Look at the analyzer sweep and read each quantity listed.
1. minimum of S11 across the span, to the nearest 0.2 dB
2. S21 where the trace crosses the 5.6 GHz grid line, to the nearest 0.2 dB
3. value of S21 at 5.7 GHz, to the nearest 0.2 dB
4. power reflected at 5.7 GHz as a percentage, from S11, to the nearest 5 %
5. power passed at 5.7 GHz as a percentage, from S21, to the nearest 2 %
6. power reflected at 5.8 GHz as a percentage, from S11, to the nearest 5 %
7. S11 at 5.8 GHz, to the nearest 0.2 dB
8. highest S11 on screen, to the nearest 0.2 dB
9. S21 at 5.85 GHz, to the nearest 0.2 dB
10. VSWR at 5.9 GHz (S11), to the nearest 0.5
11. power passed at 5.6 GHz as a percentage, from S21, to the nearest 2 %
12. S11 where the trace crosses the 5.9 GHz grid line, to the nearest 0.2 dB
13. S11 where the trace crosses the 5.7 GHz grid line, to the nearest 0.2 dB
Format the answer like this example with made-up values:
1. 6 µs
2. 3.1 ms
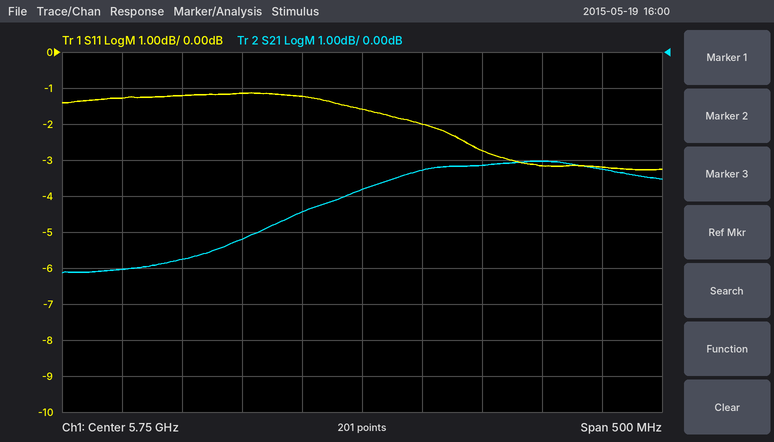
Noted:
1. -3.2 dB
2. -5.8 dB
3. -4.4 dB
4. 75 %
5. 36 %
6. 65 %
7. -2.0 dB
8. -1.2 dB
9. -3.2 dB
10. 5.5
11. 26 %
12. -3.2 dB
13. -1.2 dB
